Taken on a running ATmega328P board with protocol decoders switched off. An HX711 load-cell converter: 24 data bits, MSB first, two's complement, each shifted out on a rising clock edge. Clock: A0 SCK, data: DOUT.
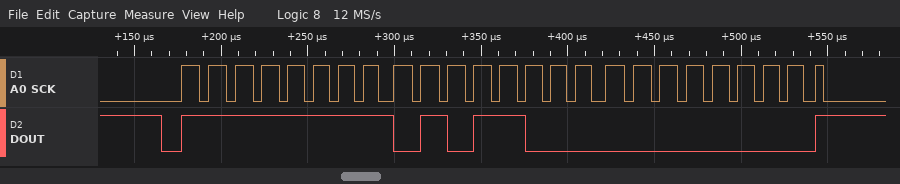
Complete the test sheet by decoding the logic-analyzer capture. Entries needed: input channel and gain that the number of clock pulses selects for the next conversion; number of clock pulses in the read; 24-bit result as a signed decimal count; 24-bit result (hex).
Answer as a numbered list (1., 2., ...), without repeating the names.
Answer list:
1. channel A, gain 128
2. 25
3. -43008
4. 0xFF5800
